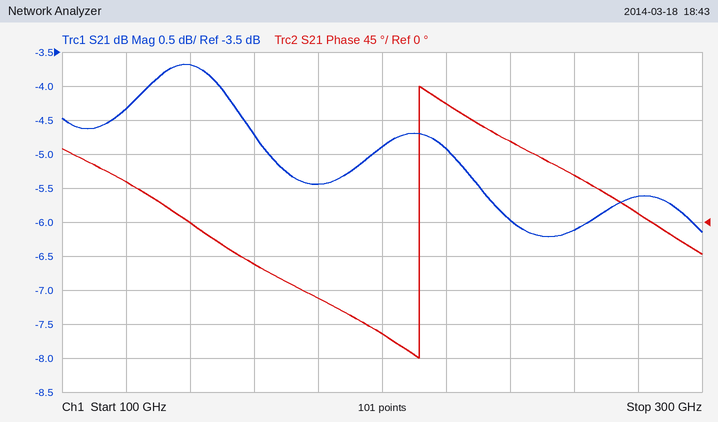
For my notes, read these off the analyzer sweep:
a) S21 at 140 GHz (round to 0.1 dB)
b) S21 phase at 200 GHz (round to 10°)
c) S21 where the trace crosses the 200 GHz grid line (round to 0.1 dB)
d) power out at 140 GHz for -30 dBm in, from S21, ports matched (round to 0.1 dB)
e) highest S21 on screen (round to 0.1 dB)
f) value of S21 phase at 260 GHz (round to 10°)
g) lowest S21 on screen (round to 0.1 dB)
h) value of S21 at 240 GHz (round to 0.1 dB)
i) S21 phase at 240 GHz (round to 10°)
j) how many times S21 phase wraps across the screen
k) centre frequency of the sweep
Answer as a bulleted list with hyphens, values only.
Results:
- -3.7 dB
- -150°
- -4.9 dB
- -33.7 dBm
- -3.7 dB
- 60°
- -6.2 dB
- -6.0 dB
- 110°
- 1
- 200 GHz
